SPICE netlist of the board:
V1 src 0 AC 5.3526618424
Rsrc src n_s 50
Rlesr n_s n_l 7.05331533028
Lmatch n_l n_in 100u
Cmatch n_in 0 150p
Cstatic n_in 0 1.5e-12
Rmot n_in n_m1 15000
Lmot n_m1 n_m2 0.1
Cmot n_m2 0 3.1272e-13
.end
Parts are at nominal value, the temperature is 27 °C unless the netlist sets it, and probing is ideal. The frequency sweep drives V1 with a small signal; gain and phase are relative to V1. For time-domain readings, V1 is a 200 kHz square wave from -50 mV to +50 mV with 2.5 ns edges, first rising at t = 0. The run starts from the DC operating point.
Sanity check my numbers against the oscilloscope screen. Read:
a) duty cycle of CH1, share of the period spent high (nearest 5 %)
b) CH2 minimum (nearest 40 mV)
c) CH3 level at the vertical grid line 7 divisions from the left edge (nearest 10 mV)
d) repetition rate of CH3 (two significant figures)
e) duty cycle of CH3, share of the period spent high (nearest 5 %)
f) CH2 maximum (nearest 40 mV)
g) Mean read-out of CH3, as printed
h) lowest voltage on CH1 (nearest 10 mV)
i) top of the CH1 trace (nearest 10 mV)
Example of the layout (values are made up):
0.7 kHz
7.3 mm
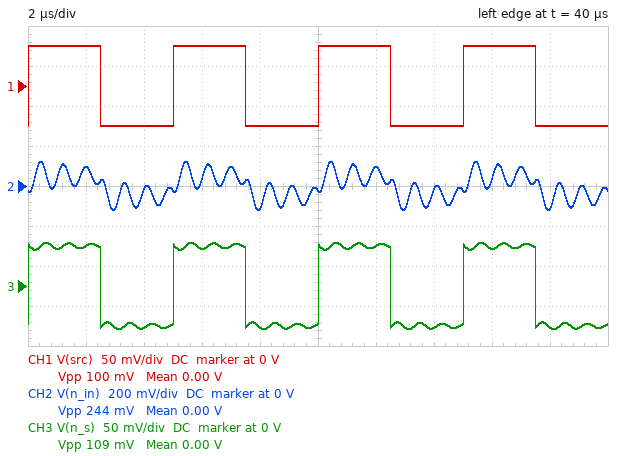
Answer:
50 %
-120 mV
-50 mV
200 kHz
50 %
120 mV
0.00 V
-50 mV
50 mV
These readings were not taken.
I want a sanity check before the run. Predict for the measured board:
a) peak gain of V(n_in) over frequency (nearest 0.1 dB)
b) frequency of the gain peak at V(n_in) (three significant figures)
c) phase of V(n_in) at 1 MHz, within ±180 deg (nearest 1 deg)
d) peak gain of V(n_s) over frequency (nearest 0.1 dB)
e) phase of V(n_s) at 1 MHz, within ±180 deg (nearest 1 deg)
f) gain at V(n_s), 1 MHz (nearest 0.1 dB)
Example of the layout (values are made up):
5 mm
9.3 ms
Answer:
23.1 dB
1.29 MHz
-8 deg
0 dB
-7 deg
-0.1 dB
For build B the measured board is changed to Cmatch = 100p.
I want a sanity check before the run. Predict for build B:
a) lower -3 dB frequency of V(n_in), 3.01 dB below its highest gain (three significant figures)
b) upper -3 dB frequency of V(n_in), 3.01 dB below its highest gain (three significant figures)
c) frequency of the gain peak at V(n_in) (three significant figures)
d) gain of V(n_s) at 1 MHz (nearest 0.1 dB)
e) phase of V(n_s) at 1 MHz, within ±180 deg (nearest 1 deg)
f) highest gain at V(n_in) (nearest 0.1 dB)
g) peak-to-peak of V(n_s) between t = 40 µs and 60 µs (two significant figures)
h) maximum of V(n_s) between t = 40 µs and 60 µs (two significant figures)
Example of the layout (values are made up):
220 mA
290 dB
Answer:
1.53 MHz
1.62 MHz
1.58 MHz
0 dB
-3 deg
24.8 dB
110 mV
53 mV
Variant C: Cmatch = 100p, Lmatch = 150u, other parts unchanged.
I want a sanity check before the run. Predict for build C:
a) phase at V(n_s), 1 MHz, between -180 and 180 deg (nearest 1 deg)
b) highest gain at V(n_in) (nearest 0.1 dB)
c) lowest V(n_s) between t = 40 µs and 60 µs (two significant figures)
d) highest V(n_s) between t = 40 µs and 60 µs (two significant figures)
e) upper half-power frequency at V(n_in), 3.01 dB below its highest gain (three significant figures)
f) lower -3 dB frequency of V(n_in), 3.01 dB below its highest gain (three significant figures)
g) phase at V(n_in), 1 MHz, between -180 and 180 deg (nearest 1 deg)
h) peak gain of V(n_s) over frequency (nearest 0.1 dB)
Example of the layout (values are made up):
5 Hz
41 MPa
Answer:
-4 deg
26.6 dB
-53 mV
53 mV
1.32 MHz
1.26 MHz
-5 deg
0 dB
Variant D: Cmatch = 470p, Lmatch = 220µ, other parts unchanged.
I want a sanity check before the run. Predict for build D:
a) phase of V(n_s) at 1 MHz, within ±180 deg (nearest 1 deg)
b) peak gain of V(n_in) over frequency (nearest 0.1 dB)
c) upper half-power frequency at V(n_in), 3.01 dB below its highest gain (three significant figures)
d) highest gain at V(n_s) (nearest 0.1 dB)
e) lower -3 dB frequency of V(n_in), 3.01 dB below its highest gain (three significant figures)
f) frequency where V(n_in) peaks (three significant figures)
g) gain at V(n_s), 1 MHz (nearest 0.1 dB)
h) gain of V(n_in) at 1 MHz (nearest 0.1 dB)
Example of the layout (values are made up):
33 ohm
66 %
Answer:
3 deg
21.6 dB
513 kHz
0 dB
472 kHz
493 kHz
0 dB
-9.8 dB
